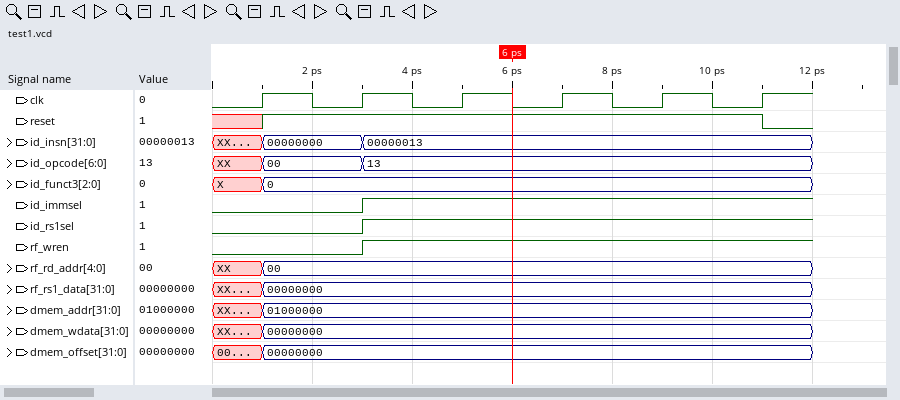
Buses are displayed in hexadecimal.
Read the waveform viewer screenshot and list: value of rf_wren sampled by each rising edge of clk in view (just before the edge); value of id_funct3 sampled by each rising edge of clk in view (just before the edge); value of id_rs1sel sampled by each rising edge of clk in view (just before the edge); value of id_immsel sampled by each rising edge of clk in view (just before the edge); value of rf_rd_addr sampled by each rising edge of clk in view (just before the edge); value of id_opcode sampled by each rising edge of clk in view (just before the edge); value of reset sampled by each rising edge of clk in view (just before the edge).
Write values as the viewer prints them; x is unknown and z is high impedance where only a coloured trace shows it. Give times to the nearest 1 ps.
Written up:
0 0 1 1 1 1
X, 0, 0, 0, 0, 0
0 0 1 1 1 1
0 0 1 1 1 1
XX, 00, 00, 00, 00, 00
XX, 00, 13, 13, 13, 13
x 1 1 1 1 1
